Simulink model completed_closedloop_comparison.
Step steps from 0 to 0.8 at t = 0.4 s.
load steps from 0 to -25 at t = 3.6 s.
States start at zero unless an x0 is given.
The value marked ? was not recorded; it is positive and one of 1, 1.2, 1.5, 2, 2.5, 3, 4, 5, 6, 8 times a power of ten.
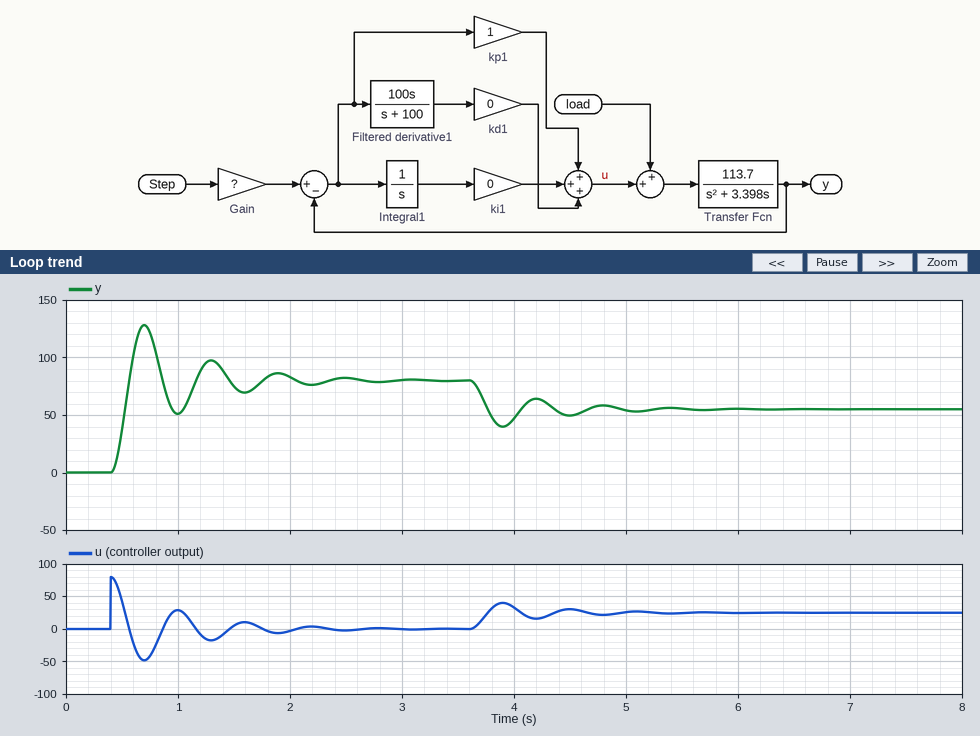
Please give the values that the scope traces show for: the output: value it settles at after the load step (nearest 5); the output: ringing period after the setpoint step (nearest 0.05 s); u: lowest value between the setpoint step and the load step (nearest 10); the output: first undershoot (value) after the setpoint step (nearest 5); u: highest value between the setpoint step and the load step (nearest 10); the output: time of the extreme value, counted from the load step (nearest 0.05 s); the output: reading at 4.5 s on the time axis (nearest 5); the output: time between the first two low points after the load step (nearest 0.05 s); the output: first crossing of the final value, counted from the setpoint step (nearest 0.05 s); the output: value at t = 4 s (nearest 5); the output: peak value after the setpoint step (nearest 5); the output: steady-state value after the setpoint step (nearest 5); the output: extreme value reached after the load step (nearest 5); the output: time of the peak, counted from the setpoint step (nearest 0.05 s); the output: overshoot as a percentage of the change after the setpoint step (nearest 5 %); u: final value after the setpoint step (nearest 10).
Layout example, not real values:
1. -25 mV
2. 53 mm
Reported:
1. 55
2. 0.60 s
3. -50
4. 50
5. 80
6. 0.30 s
7. 50
8. 0.60 s
9. 0.15 s
10. 45
11. 130
12. 80
13. 40
14. 0.30 s
15. 60 %
16. 0
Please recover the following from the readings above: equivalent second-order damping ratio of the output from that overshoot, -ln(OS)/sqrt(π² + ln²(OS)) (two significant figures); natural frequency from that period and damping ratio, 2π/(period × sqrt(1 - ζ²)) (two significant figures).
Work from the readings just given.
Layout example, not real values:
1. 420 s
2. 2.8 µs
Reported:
1. 0.16
2. 11 rad/s
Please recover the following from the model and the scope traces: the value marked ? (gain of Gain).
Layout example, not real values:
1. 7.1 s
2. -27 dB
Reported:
1. 100
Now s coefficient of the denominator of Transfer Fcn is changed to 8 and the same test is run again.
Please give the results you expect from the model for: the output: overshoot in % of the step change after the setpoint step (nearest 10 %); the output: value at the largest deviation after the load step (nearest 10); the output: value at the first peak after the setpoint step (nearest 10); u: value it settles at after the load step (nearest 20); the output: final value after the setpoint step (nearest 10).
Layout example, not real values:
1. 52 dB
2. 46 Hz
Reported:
1. 30 %
2. 50
3. 100
4. 20
5. 80
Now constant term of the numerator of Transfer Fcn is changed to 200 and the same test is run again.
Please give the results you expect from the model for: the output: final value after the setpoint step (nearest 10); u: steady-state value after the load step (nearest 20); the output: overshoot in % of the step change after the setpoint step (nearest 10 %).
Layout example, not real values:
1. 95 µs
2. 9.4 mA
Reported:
1. 80
2. 20
3. 70 %
